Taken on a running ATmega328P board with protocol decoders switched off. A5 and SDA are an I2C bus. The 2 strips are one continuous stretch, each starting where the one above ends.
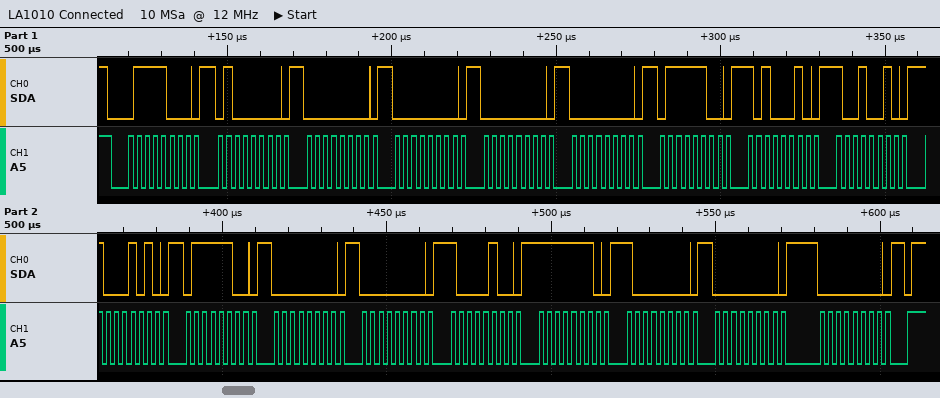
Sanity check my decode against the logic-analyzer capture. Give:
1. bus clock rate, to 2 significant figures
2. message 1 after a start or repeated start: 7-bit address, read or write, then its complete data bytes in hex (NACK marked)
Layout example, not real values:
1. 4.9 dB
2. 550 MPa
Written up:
1. 400 kHz
2. 0x3C write: 40 00 00 00 00 7C A2 92 8A 7C 00 00 84 FE 80 00 00
